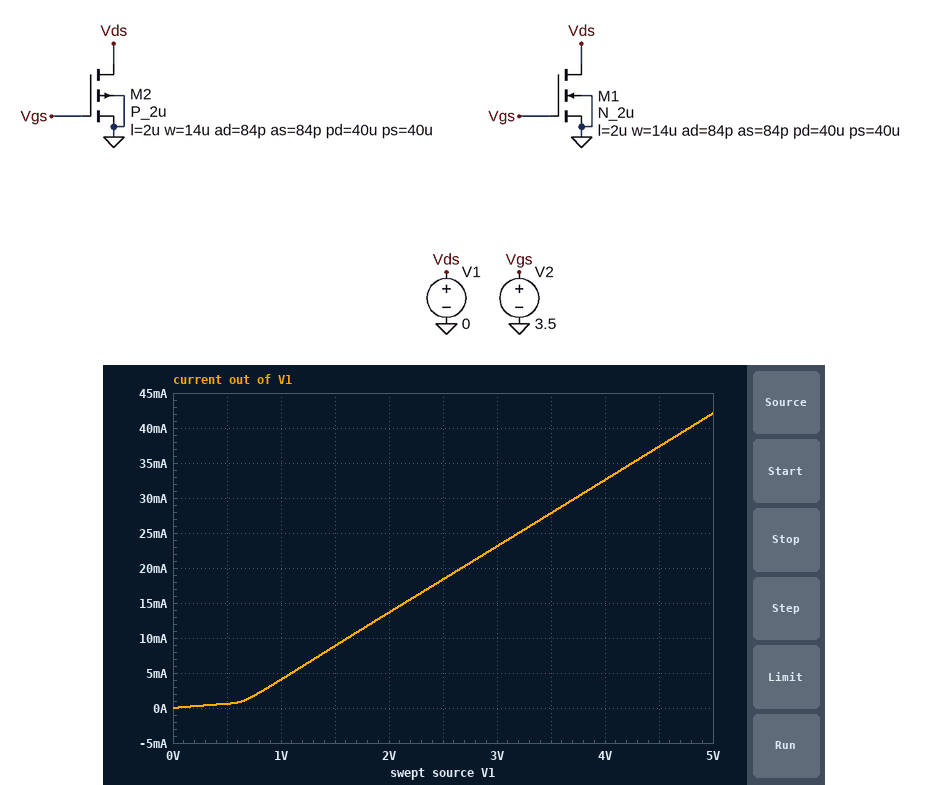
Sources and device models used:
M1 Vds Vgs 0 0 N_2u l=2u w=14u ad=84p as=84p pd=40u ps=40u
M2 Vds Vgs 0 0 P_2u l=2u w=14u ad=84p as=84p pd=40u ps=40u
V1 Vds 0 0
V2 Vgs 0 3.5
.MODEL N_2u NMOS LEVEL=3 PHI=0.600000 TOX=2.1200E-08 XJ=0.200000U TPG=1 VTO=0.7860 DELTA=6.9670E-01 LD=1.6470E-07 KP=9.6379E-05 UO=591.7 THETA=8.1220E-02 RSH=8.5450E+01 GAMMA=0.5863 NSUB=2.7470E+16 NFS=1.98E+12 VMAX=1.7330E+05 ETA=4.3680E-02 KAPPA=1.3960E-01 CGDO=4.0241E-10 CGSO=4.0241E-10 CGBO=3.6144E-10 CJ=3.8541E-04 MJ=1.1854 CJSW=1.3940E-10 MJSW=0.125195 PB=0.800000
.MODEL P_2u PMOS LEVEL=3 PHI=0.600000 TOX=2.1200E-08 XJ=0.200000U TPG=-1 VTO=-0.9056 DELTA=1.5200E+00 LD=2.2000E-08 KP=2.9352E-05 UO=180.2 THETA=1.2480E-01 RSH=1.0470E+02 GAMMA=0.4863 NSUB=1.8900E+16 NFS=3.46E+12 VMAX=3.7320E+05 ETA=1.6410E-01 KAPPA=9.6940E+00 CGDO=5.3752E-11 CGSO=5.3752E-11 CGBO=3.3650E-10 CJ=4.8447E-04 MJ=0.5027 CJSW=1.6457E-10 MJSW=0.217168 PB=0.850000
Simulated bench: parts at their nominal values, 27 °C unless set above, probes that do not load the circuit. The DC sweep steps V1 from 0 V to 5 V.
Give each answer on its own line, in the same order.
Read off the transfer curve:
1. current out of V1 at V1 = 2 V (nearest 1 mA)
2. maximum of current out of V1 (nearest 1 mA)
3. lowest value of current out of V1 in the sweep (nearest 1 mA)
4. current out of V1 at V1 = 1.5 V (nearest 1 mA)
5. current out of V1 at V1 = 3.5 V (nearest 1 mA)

14 mA
42 mA
0 A
9 mA
28 mA
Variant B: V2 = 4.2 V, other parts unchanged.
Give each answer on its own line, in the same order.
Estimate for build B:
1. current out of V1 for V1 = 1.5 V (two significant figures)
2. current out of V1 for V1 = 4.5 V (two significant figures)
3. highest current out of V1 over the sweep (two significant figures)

9.2 mA
38 mA
43 mA
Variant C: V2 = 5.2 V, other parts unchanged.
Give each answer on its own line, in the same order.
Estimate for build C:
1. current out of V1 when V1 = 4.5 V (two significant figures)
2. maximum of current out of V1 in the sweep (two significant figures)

39 mA
44 mA
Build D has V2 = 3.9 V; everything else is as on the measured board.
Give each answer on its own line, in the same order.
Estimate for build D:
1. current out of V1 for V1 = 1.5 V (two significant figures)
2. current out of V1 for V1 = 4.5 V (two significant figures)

9.1 mA
38 mA
